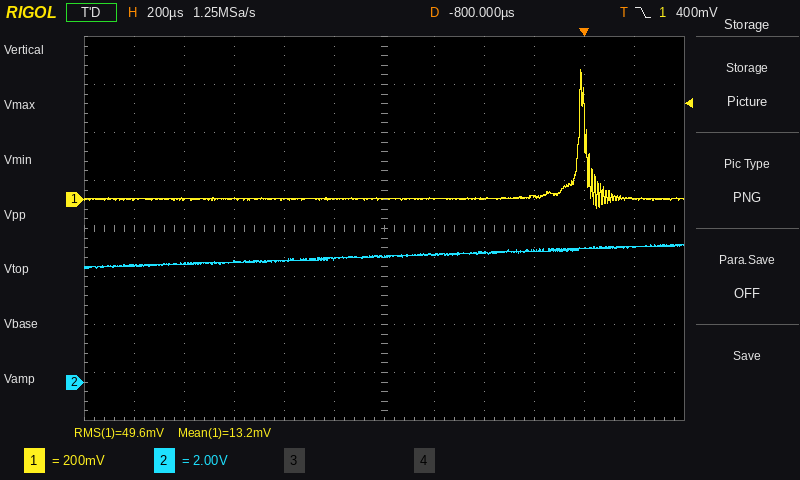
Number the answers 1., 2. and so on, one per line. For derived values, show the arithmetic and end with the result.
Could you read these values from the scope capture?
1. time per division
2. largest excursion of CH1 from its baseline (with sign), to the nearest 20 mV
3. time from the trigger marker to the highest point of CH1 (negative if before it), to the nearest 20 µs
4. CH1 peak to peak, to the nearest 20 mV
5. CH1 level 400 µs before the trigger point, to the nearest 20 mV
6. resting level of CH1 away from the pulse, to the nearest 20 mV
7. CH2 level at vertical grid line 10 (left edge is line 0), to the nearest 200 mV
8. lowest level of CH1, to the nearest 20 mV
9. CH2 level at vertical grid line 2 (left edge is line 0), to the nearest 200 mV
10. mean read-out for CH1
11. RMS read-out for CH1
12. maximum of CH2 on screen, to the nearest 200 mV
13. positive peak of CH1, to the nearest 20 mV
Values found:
1. 200 µs
2. 540 mV − (0 mV) = +540 mV
3. -20 µs
4. 540 mV − (-40 mV) = 580 mV
5. 0 mV
6. 0 mV
7. 5.6 V
8. -40 mV
9. 5.0 V
10. 13.2 mV
11. 49.6 mV
12. 5.8 V
13. 540 mV
